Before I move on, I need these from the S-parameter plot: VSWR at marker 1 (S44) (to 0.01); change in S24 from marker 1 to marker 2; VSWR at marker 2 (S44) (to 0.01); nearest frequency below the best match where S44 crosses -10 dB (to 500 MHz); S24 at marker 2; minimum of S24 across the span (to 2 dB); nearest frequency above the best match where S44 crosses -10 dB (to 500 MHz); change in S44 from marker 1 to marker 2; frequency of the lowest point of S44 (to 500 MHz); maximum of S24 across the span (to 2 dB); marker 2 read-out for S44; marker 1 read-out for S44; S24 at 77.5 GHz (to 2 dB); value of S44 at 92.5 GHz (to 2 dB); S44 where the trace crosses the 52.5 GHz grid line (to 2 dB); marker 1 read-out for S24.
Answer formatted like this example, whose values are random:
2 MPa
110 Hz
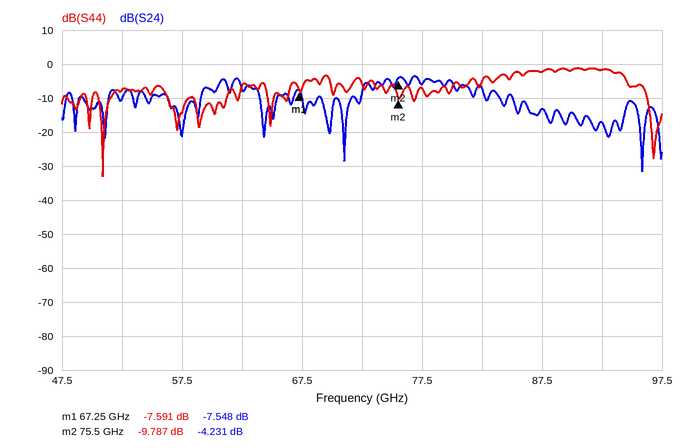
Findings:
2.43
3.317 dB
1.96
50.5 GHz
-4.231 dB
-32 dB
51.5 GHz
-2.196 dB
51.0 GHz
-4 dB
-9.787 dB
-7.591 dB
-6 dB
-2 dB
-8 dB
-7.548 dB
